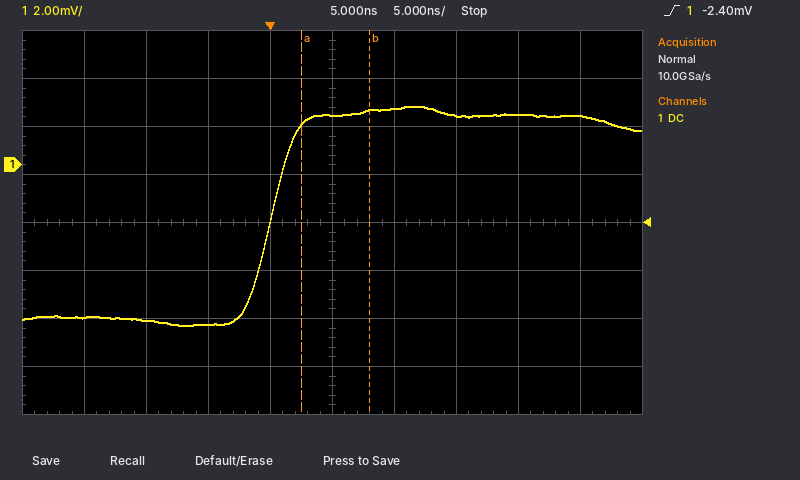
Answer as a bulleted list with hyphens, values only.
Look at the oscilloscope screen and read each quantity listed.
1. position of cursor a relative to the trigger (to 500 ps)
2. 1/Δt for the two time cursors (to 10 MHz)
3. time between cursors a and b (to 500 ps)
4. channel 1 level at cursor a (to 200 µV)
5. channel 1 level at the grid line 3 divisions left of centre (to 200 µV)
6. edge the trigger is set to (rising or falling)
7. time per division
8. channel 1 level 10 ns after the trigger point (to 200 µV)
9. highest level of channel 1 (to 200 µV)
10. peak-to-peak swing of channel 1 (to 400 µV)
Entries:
- +2.5 ns
- 180 MHz
- 5.5 ns
- 1.6 mV
- -6.4 mV
- rising
- 5 ns
- 2.4 mV
- 2.4 mV
- 9.2 mV
